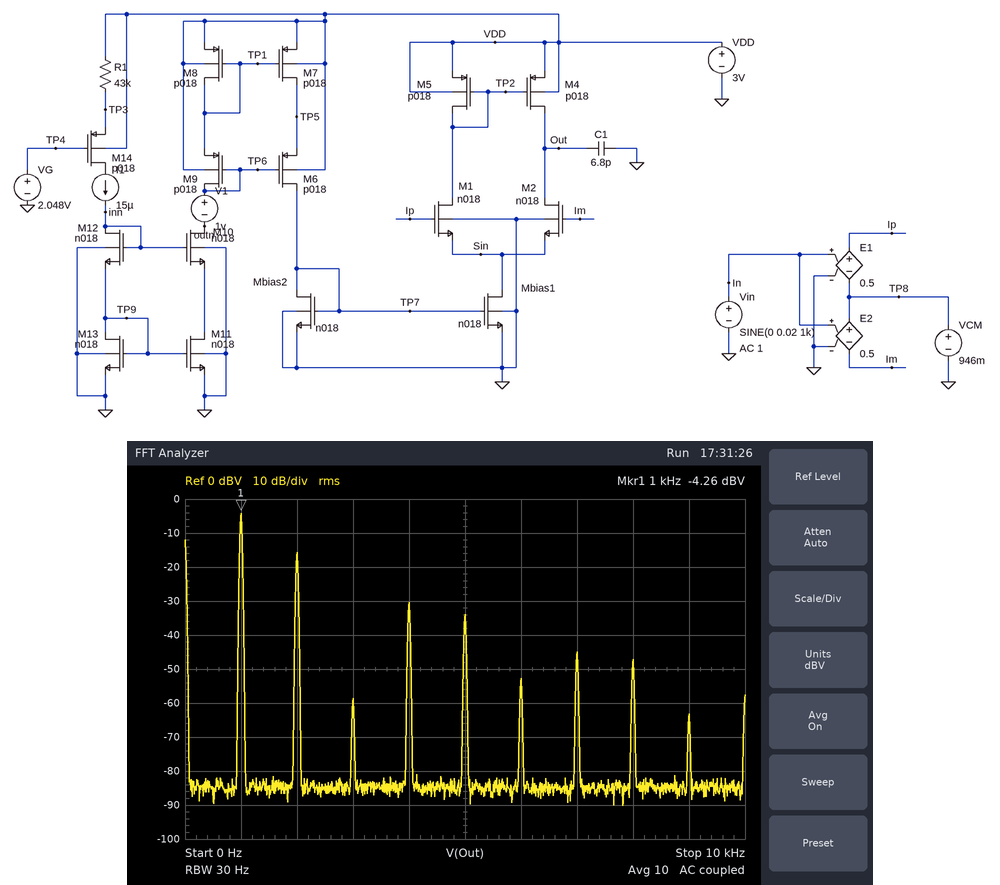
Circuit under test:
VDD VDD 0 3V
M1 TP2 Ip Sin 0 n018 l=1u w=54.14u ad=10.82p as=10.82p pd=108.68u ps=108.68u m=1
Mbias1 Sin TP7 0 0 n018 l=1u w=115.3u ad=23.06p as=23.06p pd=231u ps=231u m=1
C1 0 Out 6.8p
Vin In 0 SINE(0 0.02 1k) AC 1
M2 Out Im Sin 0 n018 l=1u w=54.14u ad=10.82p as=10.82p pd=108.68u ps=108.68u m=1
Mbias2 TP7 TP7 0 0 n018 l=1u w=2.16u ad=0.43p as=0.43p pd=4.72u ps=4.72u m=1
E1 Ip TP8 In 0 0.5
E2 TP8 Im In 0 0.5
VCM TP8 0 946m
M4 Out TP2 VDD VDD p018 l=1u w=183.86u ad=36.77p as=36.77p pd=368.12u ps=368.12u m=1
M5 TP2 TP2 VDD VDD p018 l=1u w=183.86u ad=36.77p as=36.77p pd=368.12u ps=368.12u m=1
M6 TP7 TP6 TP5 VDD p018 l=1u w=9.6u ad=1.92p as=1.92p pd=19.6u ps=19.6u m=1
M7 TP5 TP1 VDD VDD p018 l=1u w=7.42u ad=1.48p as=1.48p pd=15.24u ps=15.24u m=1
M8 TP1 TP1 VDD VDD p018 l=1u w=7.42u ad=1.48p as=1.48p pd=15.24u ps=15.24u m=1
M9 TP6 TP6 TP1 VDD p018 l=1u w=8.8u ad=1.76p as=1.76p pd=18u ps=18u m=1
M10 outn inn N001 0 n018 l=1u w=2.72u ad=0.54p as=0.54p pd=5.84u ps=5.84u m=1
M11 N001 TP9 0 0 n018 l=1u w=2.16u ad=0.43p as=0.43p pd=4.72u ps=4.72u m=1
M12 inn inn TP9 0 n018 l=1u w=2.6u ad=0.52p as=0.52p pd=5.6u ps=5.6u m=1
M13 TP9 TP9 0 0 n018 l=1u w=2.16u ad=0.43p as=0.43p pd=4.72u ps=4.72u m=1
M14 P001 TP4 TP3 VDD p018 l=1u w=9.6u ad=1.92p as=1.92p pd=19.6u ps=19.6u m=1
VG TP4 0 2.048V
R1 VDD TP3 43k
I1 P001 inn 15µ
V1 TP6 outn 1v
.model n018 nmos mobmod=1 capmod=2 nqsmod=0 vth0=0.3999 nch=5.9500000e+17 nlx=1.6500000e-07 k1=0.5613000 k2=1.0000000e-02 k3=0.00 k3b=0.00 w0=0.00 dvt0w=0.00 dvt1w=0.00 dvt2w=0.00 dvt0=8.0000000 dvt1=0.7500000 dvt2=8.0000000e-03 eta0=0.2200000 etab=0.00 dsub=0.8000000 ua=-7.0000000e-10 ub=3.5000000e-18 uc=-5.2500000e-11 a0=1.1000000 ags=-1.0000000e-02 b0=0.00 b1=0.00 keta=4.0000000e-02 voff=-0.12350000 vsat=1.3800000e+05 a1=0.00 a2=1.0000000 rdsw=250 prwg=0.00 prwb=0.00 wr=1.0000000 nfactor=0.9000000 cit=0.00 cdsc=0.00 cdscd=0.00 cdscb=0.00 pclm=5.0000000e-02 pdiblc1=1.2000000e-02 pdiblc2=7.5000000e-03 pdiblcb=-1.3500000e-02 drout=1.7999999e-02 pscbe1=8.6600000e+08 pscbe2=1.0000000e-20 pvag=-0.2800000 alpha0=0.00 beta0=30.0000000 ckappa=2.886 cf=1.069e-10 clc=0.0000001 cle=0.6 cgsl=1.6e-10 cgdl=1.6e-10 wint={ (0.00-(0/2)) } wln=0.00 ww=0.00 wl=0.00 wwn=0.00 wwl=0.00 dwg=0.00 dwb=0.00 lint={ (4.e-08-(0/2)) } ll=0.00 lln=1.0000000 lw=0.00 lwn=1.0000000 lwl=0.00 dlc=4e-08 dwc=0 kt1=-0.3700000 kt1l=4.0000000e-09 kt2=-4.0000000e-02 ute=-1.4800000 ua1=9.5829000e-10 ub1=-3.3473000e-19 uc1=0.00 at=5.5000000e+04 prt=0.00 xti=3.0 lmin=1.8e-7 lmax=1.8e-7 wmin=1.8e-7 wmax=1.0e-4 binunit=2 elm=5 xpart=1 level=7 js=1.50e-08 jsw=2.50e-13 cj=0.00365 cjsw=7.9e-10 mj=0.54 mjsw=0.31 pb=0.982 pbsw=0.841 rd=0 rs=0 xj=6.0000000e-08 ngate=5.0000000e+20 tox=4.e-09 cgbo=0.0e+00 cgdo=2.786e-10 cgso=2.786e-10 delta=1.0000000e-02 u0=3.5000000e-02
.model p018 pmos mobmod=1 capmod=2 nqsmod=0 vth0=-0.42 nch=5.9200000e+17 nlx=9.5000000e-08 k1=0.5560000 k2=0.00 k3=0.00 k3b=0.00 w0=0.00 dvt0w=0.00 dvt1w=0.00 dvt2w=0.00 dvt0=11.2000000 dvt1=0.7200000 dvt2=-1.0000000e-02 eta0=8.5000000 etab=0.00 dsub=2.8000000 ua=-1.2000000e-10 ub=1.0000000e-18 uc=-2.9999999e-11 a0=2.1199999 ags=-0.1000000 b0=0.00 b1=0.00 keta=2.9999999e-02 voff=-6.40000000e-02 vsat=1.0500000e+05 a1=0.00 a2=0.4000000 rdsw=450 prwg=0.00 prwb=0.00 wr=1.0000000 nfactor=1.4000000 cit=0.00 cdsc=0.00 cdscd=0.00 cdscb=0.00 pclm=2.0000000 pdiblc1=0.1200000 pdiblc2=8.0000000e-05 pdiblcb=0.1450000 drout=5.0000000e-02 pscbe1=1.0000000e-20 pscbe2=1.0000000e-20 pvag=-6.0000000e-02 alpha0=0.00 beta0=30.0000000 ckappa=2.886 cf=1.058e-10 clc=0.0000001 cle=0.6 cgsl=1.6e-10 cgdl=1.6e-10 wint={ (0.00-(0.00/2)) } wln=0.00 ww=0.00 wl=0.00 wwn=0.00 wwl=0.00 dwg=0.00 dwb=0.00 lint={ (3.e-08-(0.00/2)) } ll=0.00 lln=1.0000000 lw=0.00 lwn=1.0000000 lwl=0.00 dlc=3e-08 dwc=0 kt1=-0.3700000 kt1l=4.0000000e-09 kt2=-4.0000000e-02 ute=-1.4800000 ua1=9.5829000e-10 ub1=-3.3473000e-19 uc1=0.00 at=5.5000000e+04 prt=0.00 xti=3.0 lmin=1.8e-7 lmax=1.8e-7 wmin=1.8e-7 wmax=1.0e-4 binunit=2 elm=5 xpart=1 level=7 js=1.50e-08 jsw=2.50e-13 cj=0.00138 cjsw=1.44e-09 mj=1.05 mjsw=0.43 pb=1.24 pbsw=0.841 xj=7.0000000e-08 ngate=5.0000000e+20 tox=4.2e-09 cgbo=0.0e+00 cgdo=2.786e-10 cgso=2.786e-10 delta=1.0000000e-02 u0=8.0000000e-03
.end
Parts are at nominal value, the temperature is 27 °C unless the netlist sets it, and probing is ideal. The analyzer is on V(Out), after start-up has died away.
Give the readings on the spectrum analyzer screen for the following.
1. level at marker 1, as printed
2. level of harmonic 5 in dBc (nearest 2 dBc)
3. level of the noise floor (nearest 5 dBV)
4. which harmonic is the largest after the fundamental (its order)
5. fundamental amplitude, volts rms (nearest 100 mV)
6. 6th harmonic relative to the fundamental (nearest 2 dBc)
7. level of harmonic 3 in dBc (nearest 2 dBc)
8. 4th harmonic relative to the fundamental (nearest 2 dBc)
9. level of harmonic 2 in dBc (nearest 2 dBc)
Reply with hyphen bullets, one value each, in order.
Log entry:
- -4.26 dBV
- -30 dBc
- -85 dBV
- 2
- 600 mV
- -48 dBc
- -54 dBc
- -26 dBc
- -12 dBc
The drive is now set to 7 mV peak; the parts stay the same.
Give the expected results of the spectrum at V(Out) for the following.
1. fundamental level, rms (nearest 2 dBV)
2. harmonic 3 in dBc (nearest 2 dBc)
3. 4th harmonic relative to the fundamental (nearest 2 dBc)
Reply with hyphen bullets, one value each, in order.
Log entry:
- -14 dBV
- -32 dBc
- -48 dBc
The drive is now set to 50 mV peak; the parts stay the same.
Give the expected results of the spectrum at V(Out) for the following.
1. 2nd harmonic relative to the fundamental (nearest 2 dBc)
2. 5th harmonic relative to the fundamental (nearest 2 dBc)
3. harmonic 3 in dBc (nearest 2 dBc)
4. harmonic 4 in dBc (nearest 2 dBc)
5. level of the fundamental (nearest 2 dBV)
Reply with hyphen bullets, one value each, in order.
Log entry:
- -16 dBc
- -28 dBc
- -14 dBc
- -20 dBc
- 0 dBV
